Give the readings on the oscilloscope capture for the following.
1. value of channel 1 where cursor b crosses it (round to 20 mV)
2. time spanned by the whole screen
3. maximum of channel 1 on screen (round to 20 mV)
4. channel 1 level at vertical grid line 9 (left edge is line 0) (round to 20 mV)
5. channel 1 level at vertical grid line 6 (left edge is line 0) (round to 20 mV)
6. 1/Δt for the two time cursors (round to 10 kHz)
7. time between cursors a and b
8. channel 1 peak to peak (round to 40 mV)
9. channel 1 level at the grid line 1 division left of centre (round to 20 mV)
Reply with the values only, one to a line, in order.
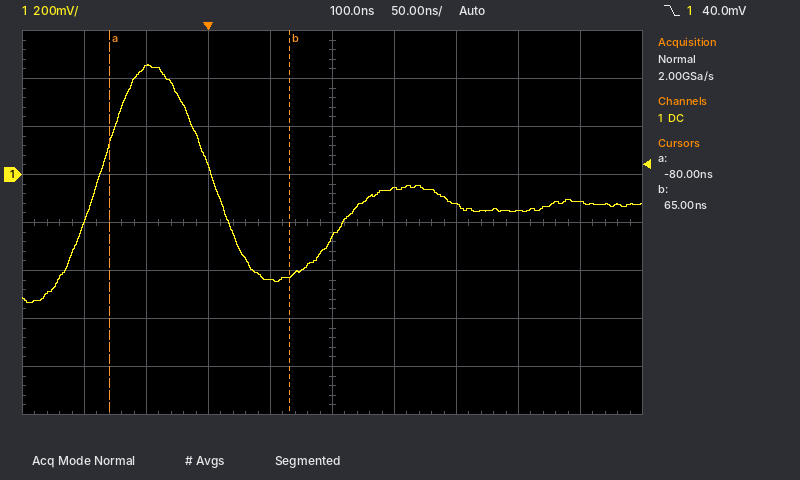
-420 mV
500 ns
460 mV
-120 mV
-60 mV
6.90 MHz
145 ns
1.00 V
-440 mV
